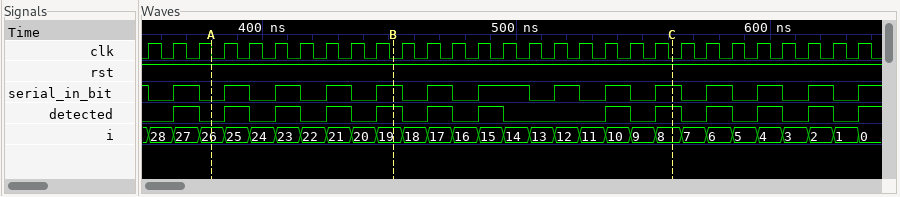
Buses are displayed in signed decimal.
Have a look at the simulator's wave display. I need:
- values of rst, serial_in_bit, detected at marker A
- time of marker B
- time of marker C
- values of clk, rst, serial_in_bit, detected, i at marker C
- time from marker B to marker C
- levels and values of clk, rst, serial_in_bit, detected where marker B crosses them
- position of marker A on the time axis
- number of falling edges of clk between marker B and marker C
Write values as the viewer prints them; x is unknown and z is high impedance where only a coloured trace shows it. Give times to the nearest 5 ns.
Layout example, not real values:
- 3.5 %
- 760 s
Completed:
- rst=1, serial_in_bit=0, detected=0
- 450 ns
- 560 ns
- clk=0, rst=1, serial_in_bit=1, detected=1, i=8
- 110 ns
- clk=0, rst=1, serial_in_bit=1, detected=1
- 380 ns
- 11
